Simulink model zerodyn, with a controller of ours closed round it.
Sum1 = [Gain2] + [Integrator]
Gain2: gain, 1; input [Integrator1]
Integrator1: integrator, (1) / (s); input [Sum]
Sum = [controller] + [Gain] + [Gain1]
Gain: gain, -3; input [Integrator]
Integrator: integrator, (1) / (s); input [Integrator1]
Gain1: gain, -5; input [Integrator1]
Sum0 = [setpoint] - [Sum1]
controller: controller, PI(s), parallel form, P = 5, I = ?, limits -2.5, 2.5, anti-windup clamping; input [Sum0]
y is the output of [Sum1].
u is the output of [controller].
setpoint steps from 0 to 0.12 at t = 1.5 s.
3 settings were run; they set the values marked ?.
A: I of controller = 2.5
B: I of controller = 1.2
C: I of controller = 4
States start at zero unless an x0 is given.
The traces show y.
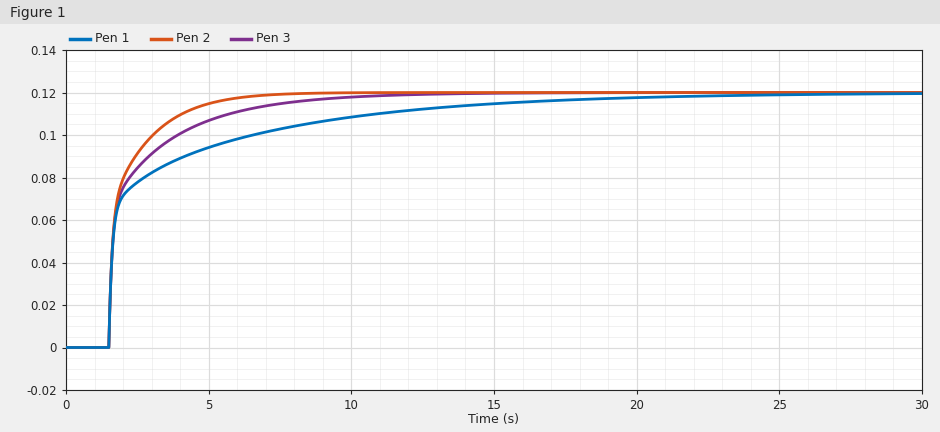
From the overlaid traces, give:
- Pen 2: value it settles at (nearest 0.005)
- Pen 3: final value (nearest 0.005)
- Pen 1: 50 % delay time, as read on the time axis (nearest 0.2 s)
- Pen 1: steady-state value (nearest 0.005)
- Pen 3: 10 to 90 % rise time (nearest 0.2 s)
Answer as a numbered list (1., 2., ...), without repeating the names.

1. 0.120
2. 0.120
3. 1.8 s
4. 0.120
5. 3.8 s
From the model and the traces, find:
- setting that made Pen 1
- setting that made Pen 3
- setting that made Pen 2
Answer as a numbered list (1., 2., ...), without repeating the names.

1. B
2. A
3. C
